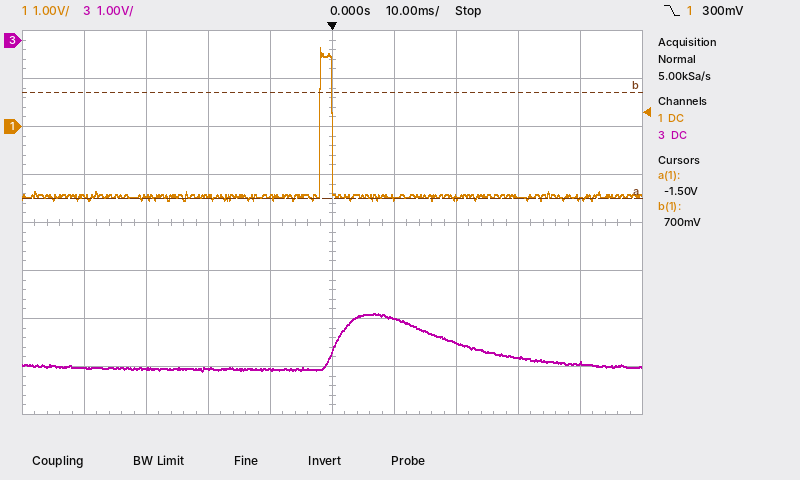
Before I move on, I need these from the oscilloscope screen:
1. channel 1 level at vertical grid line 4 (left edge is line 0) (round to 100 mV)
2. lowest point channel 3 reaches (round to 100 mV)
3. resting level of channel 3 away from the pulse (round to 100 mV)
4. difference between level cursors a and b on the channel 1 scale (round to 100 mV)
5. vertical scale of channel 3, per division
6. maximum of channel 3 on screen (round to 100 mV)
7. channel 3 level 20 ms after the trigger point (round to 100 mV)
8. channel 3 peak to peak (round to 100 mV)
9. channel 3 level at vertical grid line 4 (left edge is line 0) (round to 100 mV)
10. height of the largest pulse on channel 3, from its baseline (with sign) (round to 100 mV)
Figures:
-1.5 V
-6.9 V
-6.8 V
2.2 V
1 V
-5.7 V
-6.3 V
1.2 V
-6.9 V
+1.1 V
